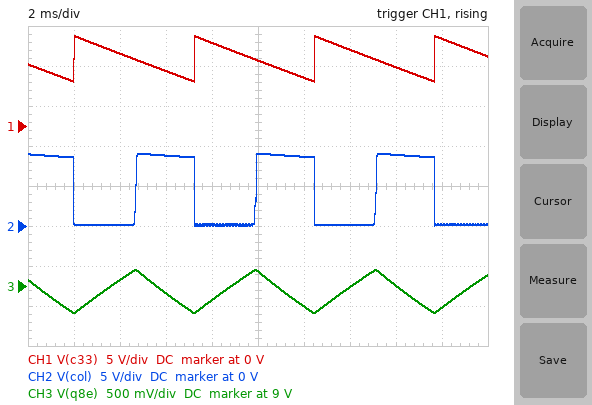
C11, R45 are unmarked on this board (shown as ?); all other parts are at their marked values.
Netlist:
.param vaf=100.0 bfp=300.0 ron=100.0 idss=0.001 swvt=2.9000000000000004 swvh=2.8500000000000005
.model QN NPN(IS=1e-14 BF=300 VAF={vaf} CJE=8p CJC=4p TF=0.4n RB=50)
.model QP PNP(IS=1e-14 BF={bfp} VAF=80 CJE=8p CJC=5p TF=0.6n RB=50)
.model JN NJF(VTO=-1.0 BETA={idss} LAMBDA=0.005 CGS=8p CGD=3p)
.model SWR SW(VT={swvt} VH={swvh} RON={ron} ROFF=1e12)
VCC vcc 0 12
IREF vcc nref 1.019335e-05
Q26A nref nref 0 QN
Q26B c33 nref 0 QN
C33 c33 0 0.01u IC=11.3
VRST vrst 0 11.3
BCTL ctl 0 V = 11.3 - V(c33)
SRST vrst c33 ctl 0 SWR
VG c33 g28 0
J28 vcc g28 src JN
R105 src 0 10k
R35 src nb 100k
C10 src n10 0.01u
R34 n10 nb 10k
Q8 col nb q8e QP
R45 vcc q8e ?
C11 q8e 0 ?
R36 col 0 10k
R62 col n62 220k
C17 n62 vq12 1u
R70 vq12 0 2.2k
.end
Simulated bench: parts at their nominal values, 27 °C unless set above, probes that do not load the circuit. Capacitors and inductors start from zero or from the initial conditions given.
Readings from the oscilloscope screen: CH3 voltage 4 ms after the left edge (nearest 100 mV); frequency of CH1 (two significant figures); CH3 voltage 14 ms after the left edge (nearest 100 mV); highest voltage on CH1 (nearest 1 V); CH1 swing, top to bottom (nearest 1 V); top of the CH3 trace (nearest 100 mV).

9.1 V
190 Hz
9.0 V
11 V
6 V
9.2 V
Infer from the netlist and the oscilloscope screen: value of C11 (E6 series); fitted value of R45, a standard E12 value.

2.2 µF
6.8 kΩ
